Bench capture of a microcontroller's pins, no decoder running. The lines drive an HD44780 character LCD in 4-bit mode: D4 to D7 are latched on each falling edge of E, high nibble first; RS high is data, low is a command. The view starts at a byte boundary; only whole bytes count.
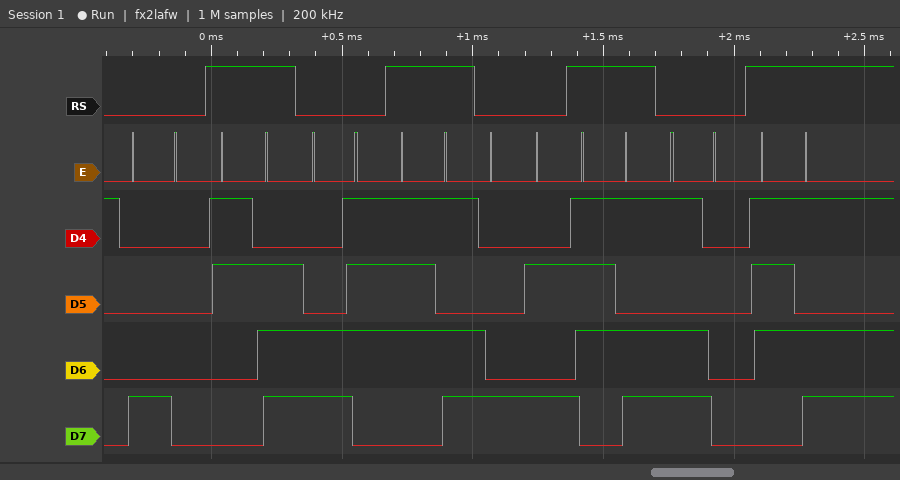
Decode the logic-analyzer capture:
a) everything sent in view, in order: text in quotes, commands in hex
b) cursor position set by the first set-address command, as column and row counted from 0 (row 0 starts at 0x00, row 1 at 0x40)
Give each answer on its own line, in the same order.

0x80 ">" 0xC7 "}" 0x8A "}" 0xD0 "}"
column 0, row 0
